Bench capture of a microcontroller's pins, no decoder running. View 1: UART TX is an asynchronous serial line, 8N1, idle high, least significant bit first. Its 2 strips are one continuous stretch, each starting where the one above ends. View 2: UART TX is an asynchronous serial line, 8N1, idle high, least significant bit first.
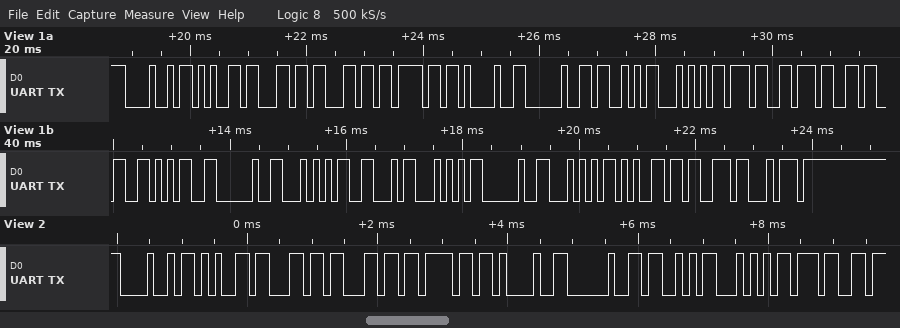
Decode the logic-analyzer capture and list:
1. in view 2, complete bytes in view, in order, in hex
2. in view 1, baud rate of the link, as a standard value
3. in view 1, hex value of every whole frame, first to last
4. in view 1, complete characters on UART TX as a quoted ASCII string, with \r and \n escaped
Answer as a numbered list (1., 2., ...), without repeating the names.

1. 0x48 0x65 0x6C 0x6C 0x6F 0x21 0x20 0x53 0x54 0x37
2. 9600 baud
3. 48 65 6C 6C 6F 21 20 53 54 37 37 33 35 20 54 46 54 20 54 65 73 74
4. "Hello! ST7735 TFT Test"
